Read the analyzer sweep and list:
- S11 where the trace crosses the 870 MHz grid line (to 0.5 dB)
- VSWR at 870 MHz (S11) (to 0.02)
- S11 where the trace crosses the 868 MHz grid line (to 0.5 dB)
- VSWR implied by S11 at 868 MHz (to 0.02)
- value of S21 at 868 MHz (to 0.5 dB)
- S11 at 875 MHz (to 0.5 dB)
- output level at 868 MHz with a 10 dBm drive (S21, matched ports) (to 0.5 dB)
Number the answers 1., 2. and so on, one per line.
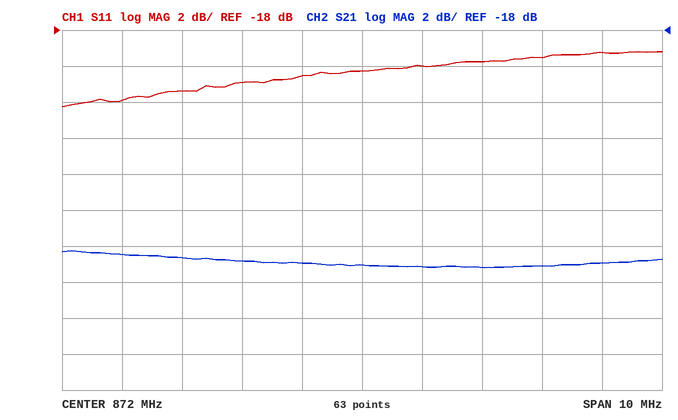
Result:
1. -21.0 dB
2. 1.20
3. -22.0 dB
4. 1.18
5. -30.5 dB
6. -19.5 dB
7. -20.5 dBm
